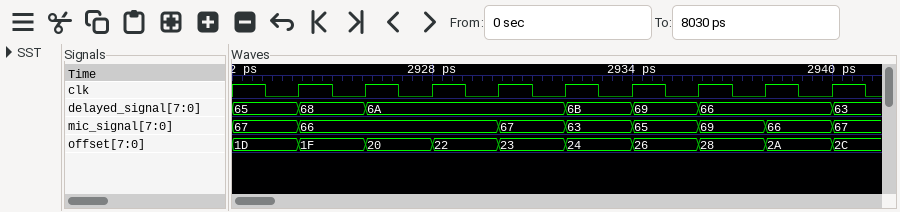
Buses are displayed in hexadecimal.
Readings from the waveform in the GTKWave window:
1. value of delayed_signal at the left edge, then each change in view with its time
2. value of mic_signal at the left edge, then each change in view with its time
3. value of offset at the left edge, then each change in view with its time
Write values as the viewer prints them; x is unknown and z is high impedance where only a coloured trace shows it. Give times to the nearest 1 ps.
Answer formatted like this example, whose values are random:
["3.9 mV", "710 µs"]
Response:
["65, 68 at 2924 ps, 6A at 2926 ps, 6B at 2932 ps, 69 at 2934 ps, 66 at 2936 ps, 63 at 2940 ps", "67, 66 at 2924 ps, 67 at 2930 ps, 63 at 2932 ps, 65 at 2934 ps, 69 at 2936 ps, 66 at 2938 ps, 67 at 2940 ps", "1D, 1F at 2924 ps, 20 at 2926 ps, 22 at 2928 ps, 23 at 2930 ps, 24 at 2932 ps, 26 at 2934 ps, 28 at 2936 ps, 2A at 2938 ps, 2C at 2940 ps"]
